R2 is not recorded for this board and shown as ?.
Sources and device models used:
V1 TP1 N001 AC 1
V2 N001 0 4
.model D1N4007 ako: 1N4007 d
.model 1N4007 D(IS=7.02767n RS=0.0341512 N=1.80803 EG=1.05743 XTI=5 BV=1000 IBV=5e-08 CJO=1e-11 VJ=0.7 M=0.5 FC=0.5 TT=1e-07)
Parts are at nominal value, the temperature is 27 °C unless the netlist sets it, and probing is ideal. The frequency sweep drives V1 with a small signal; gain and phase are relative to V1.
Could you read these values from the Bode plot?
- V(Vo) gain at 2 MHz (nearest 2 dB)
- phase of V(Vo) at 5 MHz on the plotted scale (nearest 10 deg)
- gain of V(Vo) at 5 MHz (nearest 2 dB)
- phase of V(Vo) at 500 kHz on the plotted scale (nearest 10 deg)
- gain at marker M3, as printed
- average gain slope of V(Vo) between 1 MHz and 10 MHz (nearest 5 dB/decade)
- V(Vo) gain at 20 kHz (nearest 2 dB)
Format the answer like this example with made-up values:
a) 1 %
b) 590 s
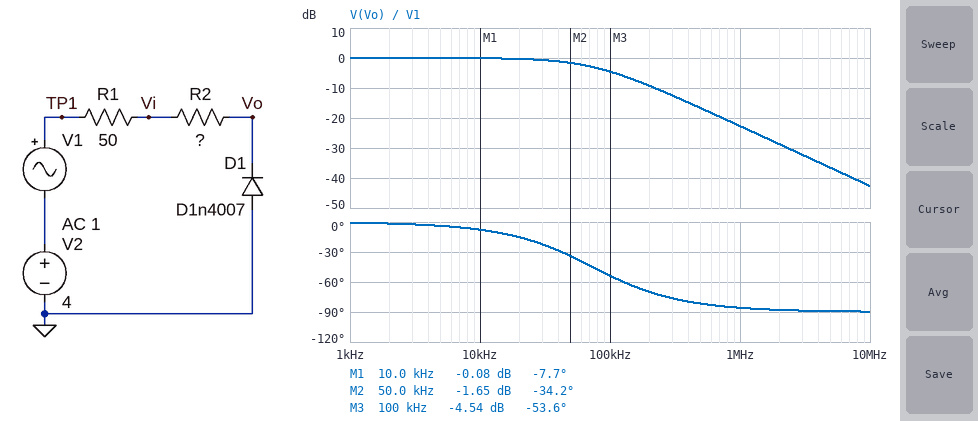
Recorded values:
a) -28 dB
b) -90 deg
c) -36 dB
d) -80 deg
e) -4.54 dB
f) -20 dB/decade
g) 0 dB
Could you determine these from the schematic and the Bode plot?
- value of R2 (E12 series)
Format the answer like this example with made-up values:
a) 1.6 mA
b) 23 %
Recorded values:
a) 560 kΩ
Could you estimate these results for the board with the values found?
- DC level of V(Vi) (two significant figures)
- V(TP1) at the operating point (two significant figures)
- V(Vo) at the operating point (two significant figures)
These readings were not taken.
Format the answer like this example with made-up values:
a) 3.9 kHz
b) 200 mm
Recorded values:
a) 4.0 V
b) 4.0 V
c) 4.0 V
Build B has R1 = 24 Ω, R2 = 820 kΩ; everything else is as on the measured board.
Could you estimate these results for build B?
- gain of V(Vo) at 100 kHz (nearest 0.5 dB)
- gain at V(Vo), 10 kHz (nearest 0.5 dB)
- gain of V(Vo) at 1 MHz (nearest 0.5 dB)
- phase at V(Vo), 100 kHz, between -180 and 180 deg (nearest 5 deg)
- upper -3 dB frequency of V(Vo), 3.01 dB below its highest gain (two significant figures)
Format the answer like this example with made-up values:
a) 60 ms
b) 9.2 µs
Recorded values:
a) -7.0 dB
b) 0 dB
c) -26.0 dB
d) -65 deg
e) 50 kHz
